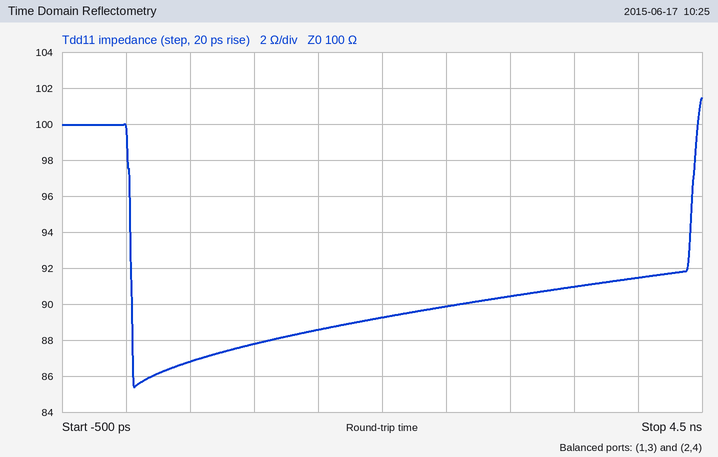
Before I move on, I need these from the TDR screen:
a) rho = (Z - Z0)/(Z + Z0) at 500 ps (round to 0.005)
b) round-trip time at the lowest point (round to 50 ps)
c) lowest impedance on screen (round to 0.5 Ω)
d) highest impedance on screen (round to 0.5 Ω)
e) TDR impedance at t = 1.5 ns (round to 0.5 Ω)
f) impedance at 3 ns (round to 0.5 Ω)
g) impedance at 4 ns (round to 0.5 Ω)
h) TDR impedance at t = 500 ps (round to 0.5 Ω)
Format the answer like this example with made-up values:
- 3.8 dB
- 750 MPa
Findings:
- -0.070
- 50 ps
- 85.5 Ω
- 101.5 Ω
- 88.5 Ω
- 90.5 Ω
- 91.5 Ω
- 87.0 Ω
